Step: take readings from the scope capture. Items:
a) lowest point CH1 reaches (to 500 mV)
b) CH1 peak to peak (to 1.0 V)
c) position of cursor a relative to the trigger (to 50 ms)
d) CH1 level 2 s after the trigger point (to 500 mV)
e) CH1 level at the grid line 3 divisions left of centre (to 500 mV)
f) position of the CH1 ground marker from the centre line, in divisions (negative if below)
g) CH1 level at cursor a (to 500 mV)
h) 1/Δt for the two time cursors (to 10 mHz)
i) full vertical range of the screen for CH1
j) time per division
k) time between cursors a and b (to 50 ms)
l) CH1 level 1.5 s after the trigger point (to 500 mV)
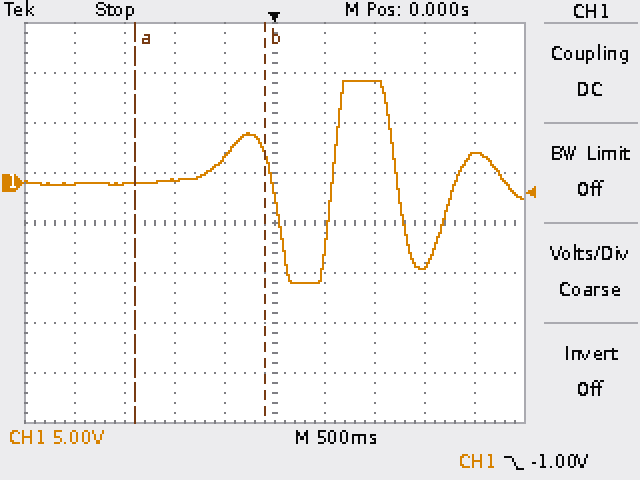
-10.0 V
20.0 V
-1.40 s
3.0 V
0.0 V
+0.8 div
0.0 V
770 mHz
40 V
500 ms
1.30 s
-8.5 V
